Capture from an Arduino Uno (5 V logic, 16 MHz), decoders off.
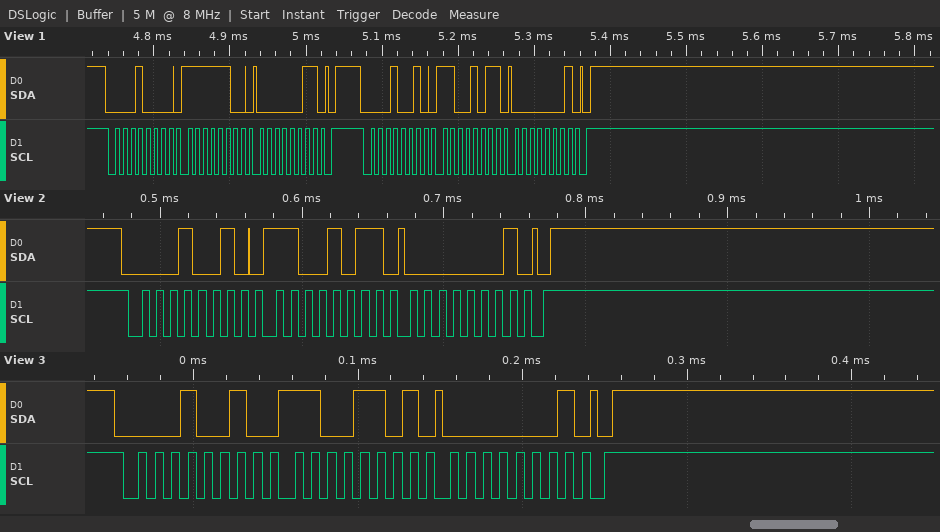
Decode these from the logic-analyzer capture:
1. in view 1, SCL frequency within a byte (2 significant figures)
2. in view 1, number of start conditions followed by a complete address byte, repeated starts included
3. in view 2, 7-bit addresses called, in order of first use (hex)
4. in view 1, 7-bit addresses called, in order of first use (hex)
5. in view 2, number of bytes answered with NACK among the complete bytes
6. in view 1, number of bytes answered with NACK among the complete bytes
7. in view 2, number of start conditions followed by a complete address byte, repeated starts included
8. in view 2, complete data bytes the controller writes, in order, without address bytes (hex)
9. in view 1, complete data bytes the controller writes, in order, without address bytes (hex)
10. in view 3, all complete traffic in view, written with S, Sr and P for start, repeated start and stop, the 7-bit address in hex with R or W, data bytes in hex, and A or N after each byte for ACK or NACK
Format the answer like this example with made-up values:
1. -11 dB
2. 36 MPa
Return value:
1. 100 kHz
2. 2
3. 0x09
4. 0x08 0x09
5. 0
6. 0
7. 1
8. CB 01
9. FC 03 CB 01
10. S 09W A CD A 01 A P
